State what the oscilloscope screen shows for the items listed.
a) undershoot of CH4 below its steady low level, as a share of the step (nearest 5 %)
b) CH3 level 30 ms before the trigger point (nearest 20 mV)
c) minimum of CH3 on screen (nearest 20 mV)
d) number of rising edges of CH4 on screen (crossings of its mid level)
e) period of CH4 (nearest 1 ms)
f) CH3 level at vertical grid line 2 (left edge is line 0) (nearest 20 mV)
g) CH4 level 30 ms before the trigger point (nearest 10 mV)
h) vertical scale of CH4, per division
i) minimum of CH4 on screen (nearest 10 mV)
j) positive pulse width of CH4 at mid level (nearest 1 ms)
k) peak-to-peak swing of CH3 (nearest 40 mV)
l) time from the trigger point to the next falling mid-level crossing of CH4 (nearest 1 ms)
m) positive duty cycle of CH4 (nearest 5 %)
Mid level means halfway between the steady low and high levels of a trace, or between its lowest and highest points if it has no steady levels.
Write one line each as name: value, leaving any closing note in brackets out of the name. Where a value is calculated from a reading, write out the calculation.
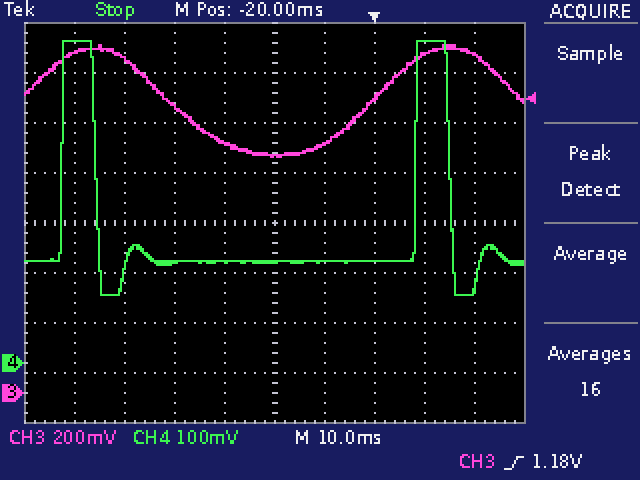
undershoot of CH4 below its steady low level, as a share of the step: 15 %
CH3 level 30 ms before the trigger point: 1.00 V
minimum of CH3 on screen: 940 mV
number of rising edges of CH4 on screen: 2
period of CH4: 71 ms
CH3 level at vertical grid line 2 (left edge is line 0): 1.34 V
CH4 level 30 ms before the trigger point: 200 mV
vertical scale of CH4, per division: 100 mV
minimum of CH4 on screen: 140 mV
positive pulse width of CH4 at mid level: 7 ms
peak-to-peak swing of CH3: 440 mV
time from the trigger point to the next falling mid-level crossing of CH4: 15 ms
positive duty cycle of CH4: 7 ms / 71 ms ≈ 10 %
